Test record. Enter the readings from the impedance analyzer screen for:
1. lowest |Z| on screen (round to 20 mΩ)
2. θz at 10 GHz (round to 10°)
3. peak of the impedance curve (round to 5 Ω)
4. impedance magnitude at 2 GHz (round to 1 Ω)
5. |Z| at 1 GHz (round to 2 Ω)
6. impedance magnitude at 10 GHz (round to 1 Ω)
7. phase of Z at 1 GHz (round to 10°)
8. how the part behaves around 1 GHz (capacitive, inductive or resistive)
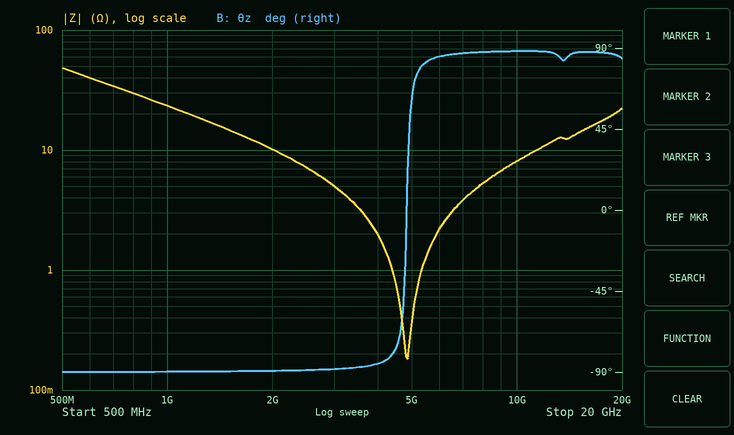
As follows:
180 mΩ
90°
50 Ω
10 Ω
24 Ω
8 Ω
-90°
capacitive
